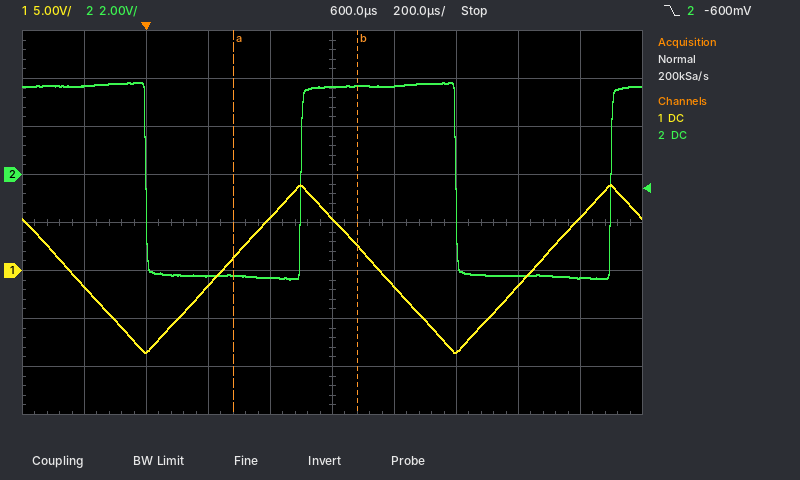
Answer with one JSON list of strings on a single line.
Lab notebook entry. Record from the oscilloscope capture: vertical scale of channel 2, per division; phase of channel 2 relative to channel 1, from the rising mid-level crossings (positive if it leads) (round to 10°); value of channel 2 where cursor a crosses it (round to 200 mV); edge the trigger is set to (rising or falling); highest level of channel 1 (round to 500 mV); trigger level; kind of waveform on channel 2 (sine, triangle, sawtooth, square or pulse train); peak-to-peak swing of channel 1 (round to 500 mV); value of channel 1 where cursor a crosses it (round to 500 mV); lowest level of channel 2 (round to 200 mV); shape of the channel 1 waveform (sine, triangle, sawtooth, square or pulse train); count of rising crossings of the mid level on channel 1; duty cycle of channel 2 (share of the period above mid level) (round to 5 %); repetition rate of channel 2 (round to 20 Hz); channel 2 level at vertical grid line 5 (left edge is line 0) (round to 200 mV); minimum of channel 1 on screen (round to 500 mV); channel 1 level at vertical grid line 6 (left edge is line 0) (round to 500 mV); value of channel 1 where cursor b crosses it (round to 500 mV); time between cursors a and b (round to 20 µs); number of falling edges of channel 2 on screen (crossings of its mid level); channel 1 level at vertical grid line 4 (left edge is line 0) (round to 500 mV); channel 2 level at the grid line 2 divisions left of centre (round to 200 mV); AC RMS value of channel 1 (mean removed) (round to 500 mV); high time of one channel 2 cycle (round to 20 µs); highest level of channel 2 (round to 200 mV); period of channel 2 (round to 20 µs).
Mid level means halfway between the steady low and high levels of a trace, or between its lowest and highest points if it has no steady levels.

["2 V", "-90°", "-4.2 V", "falling", "9.0 V", "-600 mV", "square", "17.5 V", "1.5 V", "-4.4 V", "triangle", "2", "50 %", "1.00 kHz", "3.6 V", "-8.5 V", "-1.5 V", "2.5 V", "400 µs", "2", "5.5 V", "-4.2 V", "5.0 V", "500 µs", "3.8 V", "1.00 ms"]
